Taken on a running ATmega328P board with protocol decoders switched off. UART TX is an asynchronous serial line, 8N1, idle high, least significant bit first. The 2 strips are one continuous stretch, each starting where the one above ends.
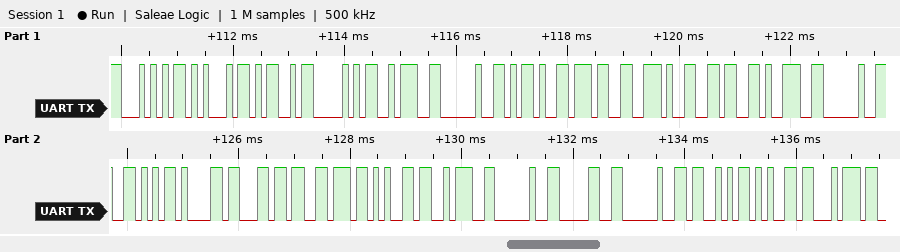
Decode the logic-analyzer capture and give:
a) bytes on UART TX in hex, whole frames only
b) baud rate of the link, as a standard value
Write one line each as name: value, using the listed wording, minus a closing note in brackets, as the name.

bytes on UART TX in hex, whole frames only: 54 45 4D 50 3A 20 2D 37 2E 36 39 20 56 61 6C 76 65 3A 20 30 20 53 65 74
baud rate of the link, as a standard value: 9600 baud
